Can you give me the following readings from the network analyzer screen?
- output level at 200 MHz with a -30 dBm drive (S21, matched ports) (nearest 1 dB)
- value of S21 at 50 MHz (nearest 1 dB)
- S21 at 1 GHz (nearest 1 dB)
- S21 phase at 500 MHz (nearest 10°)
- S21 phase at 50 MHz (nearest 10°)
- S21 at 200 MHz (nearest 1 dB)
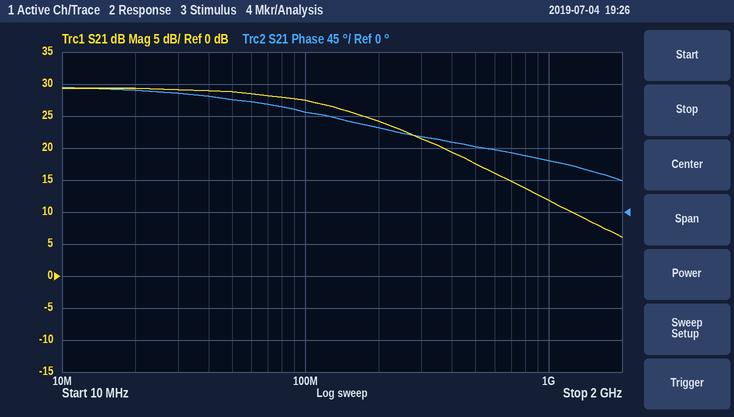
-6 dBm
29 dB
12 dB
90°
160°
24 dB
